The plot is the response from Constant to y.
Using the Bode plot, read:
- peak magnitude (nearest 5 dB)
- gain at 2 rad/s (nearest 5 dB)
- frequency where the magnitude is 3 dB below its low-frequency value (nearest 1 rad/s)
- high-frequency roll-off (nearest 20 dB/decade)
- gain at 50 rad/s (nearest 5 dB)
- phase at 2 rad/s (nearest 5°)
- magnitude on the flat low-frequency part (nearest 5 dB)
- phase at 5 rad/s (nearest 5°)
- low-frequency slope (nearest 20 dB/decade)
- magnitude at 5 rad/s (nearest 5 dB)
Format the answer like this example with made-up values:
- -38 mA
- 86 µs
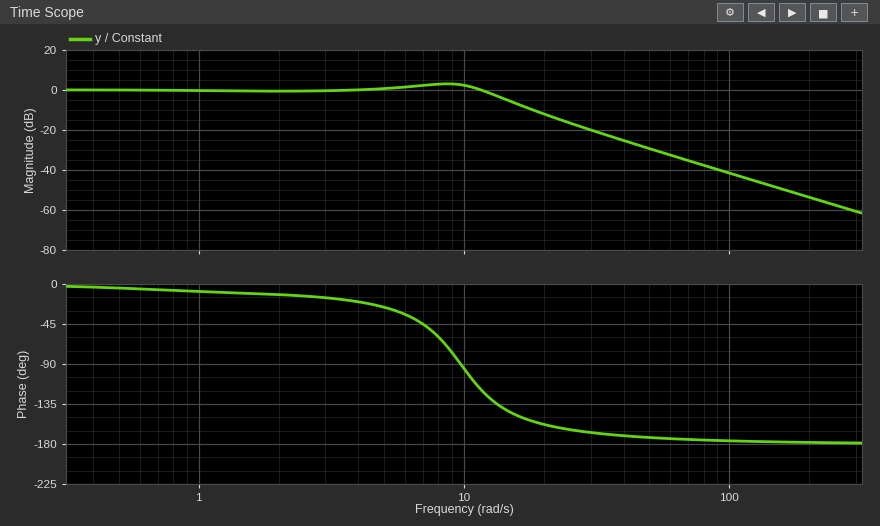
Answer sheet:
- 5 dB
- 0 dB
- 13 rad/s
- -40 dB/decade
- -30 dB
- -10°
- 0 dB
- -25°
- 0 dB/decade
- 0 dB
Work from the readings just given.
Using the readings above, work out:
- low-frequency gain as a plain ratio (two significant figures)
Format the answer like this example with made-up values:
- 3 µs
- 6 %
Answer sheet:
- 1.0
